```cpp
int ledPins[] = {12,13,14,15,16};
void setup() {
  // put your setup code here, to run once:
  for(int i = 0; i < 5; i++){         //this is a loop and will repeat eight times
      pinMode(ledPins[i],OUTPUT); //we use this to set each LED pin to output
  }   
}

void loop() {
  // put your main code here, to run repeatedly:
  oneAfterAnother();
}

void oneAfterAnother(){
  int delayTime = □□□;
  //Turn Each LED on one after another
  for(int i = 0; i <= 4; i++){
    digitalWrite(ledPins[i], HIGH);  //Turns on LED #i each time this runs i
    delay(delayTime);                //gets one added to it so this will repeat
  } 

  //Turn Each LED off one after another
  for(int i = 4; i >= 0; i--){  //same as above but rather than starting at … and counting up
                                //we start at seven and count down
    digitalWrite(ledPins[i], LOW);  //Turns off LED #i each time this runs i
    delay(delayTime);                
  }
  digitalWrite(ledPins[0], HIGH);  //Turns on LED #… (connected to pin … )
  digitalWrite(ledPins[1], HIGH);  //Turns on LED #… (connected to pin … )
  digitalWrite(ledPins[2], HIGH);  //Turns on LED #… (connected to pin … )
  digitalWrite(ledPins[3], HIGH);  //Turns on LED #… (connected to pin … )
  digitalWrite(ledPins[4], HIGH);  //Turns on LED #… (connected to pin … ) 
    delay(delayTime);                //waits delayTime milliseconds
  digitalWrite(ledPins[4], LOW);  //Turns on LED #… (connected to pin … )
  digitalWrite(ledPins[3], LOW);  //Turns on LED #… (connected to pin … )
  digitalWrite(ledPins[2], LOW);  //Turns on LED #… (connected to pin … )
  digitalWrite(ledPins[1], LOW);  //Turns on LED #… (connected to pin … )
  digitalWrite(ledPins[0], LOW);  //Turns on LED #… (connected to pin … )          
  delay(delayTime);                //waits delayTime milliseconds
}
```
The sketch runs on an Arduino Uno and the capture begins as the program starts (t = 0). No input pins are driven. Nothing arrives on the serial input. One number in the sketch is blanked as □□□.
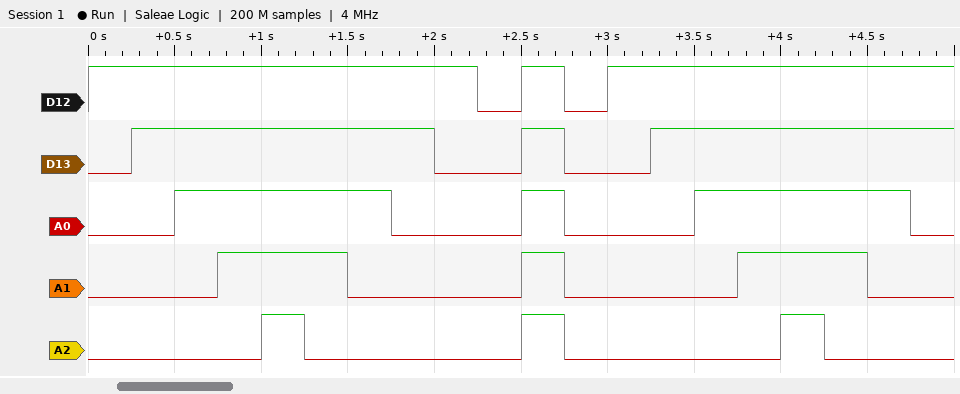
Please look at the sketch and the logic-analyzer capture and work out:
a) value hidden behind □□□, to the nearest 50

250
